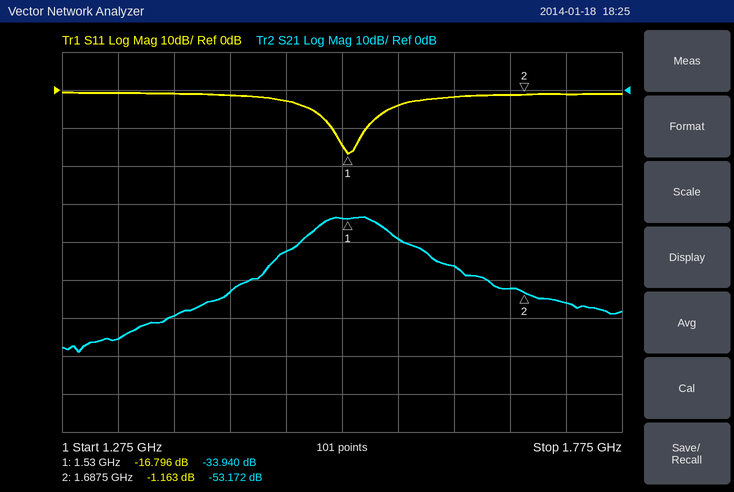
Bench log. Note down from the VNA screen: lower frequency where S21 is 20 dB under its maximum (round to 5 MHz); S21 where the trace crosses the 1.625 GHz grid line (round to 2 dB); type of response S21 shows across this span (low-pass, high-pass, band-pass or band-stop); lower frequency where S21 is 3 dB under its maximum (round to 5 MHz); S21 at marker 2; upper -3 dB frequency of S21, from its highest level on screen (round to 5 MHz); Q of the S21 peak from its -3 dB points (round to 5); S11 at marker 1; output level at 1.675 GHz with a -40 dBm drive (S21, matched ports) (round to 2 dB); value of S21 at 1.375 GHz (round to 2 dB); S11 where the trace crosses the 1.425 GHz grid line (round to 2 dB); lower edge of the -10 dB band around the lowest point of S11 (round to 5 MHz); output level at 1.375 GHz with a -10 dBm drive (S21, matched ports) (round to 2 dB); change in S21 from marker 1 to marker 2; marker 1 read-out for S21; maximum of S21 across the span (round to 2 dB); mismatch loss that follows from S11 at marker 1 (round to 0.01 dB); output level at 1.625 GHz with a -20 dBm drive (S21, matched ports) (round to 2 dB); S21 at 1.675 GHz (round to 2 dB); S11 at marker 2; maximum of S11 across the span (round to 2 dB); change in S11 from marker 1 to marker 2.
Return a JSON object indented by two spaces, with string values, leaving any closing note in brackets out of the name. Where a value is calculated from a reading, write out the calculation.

{
  "lower frequency where S21 is 20 dB under its maximum": "1.425 GHz",
  "S21 where the trace crosses the 1.625 GHz grid line": "-46 dB",
  "type of response S21 shows across this span": "band-pass",
  "lower frequency where S21 is 3 dB under its maximum": "1.500 GHz",
  "S21 at marker 2": "-53.172 dB",
  "upper -3 dB frequency of S21, from its highest level on screen": "1.565 GHz",
  "Q of the S21 peak from its -3 dB points": "1.5325 GHz / 65 MHz ≈ 23.6, so 25 to the nearest 5",
  "S11 at marker 1": "-16.796 dB",
  "output level at 1.675 GHz with a -40 dBm drive (S21, matched ports)": "-40 dBm + (-52 dB) = -92 dBm",
  "value of S21 at 1.375 GHz": "-60 dB",
  "S11 where the trace crosses the 1.425 GHz grid line": "-2 dB",
  "lower edge of the -10 dB band around the lowest point of S11": "1.515 GHz",
  "output level at 1.375 GHz with a -10 dBm drive (S21, matched ports)": "-10 dBm + (-60 dB) = -70 dBm",
  "change in S21 from marker 1 to marker 2": "-53.172 − (-33.94) = -19.232 dB",
  "marker 1 read-out for S21": "-33.940 dB",
  "maximum of S21 across the span": "-34 dB",
  "mismatch loss that follows from S11 at marker 1": "−10 log10(1 − 10^(-16.796/10)) ≈ 0.09 dB",
  "output level at 1.625 GHz with a -20 dBm drive (S21, matched ports)": "-20 dBm + (-46 dB) = -66 dBm",
  "S21 at 1.675 GHz": "-52 dB",
  "S11 at marker 2": "-1.163 dB",
  "maximum of S11 across the span": "0 dB",
  "change in S11 from marker 1 to marker 2": "-1.163 − (-16.796) = 15.633 dB"
}
